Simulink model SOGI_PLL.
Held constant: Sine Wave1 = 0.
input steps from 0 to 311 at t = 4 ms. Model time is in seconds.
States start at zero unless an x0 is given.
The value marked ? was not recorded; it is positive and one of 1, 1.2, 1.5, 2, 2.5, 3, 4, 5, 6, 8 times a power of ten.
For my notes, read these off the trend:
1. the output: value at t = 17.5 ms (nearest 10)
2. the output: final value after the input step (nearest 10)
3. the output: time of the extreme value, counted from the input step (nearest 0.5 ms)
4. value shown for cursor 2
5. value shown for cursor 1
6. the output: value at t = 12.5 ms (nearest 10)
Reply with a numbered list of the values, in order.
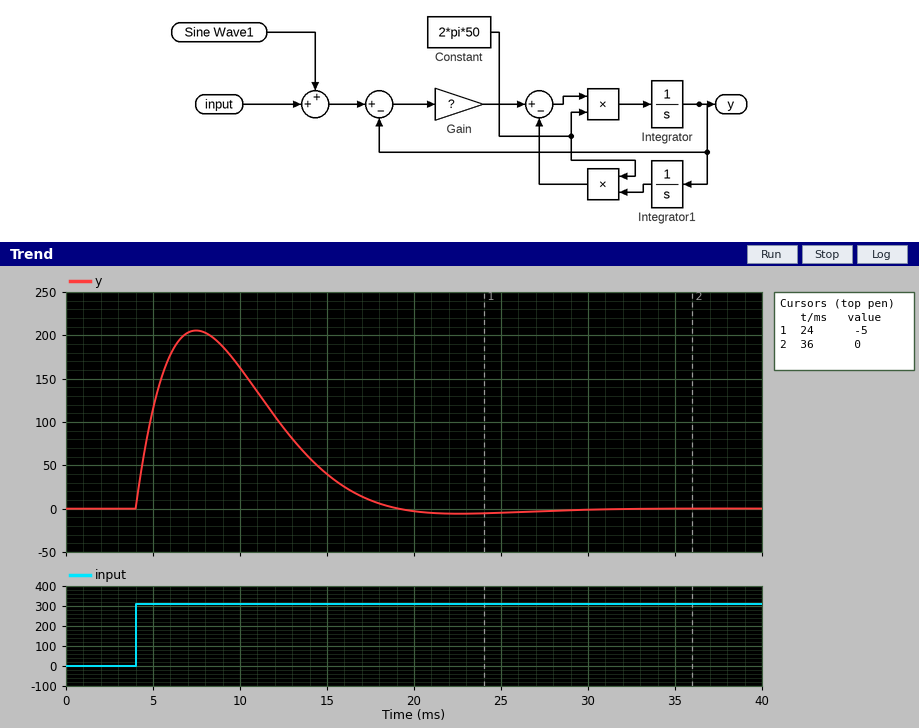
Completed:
1. 10
2. 0
3. 3.5 ms
4. 0
5. -5
6. 90
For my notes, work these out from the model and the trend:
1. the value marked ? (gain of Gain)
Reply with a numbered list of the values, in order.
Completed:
1. 1.5
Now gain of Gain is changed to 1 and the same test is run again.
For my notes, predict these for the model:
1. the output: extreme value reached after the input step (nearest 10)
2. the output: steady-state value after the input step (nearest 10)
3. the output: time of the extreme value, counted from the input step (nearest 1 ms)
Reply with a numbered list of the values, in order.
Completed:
1. 170
2. 0
3. 4 ms
